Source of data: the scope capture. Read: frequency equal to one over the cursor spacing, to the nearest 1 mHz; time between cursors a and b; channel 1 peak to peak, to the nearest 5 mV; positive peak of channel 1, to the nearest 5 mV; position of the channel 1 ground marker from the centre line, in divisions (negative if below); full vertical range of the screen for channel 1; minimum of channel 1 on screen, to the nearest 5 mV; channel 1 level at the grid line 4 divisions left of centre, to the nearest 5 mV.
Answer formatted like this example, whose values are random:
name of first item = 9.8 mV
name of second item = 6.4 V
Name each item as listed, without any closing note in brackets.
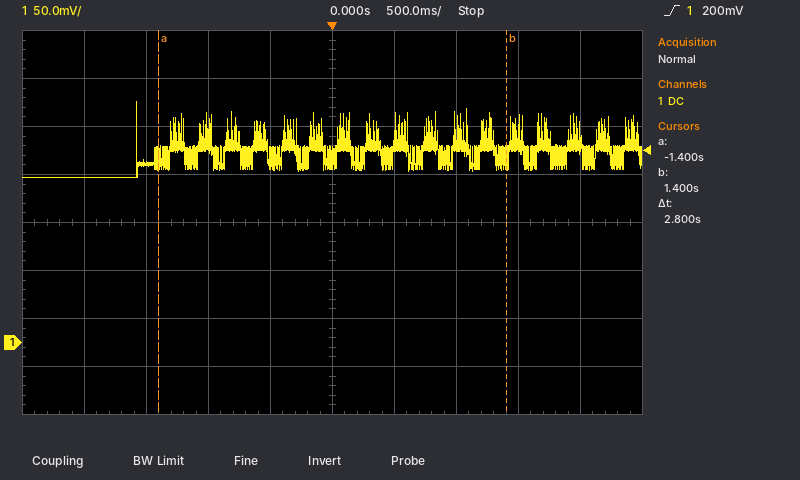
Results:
frequency equal to one over the cursor spacing, to the nearest 1 mHz = 357 mHz
time between cursors a and b = 2.8 s
channel 1 peak to peak, to the nearest 5 mV = 80 mV
positive peak of channel 1, to the nearest 5 mV = 250 mV
position of the channel 1 ground marker from the centre line, in divisions = -2.5 div
full vertical range of the screen for channel 1 = 400 mV
minimum of channel 1 on screen, to the nearest 5 mV = 170 mV
channel 1 level at the grid line 4 divisions left of centre, to the nearest 5 mV = 170 mV
